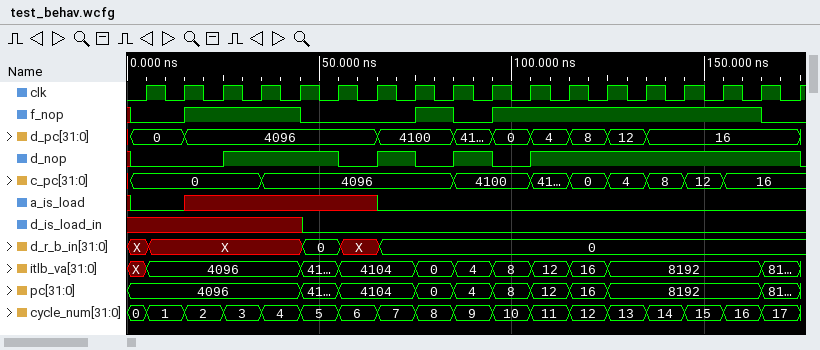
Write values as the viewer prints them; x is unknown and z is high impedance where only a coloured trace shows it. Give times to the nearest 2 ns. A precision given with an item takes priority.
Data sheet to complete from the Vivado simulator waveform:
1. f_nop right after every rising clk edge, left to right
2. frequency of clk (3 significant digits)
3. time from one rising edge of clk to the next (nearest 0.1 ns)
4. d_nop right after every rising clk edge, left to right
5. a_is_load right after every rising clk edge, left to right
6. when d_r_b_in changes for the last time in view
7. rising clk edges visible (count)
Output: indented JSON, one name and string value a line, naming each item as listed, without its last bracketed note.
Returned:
{
  "f_nop right after every rising clk edge, left to right": "0 1 1 1 0 0 0 1 0 1 1 1 1 1 1 1 0 0",
  "frequency of clk": "100 MHz",
  "time from one rising edge of clk to the next": "10 ns",
  "d_nop right after every rising clk edge, left to right": "0 0 1 1 1 0 1 0 1 0 1 1 1 1 1 1 1 0",
  "a_is_load right after every rising clk edge, left to right": "0 x x x x x 0 0 0 0 0 0 0 0 0 0 0 0",
  "when d_r_b_in changes for the last time in view": "66 ns",
  "rising clk edges visible": "18"
}
